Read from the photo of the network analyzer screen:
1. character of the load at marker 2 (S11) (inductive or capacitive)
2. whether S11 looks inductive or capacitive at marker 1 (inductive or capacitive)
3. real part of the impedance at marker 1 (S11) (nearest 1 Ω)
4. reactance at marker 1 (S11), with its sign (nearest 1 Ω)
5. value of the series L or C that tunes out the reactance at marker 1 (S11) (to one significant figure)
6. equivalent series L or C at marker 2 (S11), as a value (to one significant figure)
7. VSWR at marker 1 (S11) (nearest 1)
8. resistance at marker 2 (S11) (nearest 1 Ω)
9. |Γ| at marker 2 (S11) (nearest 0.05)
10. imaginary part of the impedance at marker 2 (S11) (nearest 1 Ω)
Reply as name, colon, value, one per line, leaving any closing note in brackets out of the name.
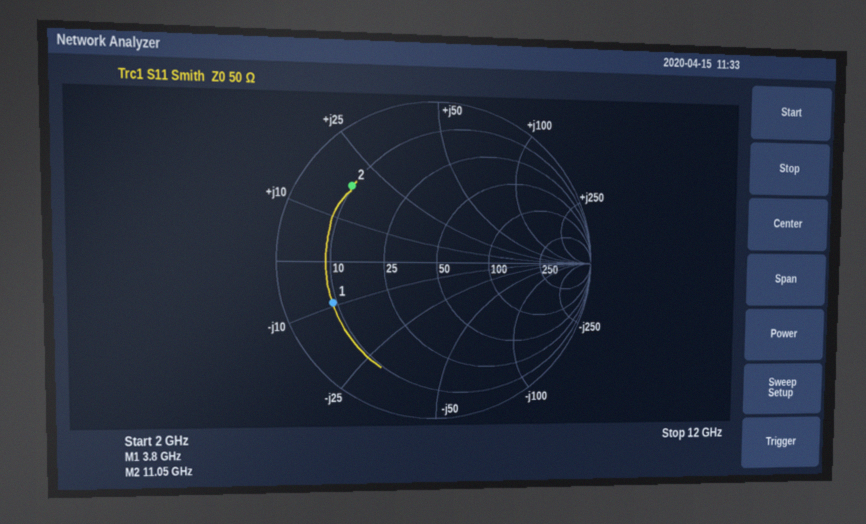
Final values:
character of the load at marker 2 (S11): inductive
whether S11 looks inductive or capacitive at marker 1: capacitive
real part of the impedance at marker 1 (S11): 9 Ω
reactance at marker 1 (S11), with its sign: -9 Ω
value of the series L or C that tunes out the reactance at marker 1 (S11): 400 pH
equivalent series L or C at marker 2 (S11), as a value: 300 pH
VSWR at marker 1 (S11): 6
resistance at marker 2 (S11): 10 Ω
|Γ| at marker 2 (S11): 0.70
imaginary part of the impedance at marker 2 (S11): +18 Ω
